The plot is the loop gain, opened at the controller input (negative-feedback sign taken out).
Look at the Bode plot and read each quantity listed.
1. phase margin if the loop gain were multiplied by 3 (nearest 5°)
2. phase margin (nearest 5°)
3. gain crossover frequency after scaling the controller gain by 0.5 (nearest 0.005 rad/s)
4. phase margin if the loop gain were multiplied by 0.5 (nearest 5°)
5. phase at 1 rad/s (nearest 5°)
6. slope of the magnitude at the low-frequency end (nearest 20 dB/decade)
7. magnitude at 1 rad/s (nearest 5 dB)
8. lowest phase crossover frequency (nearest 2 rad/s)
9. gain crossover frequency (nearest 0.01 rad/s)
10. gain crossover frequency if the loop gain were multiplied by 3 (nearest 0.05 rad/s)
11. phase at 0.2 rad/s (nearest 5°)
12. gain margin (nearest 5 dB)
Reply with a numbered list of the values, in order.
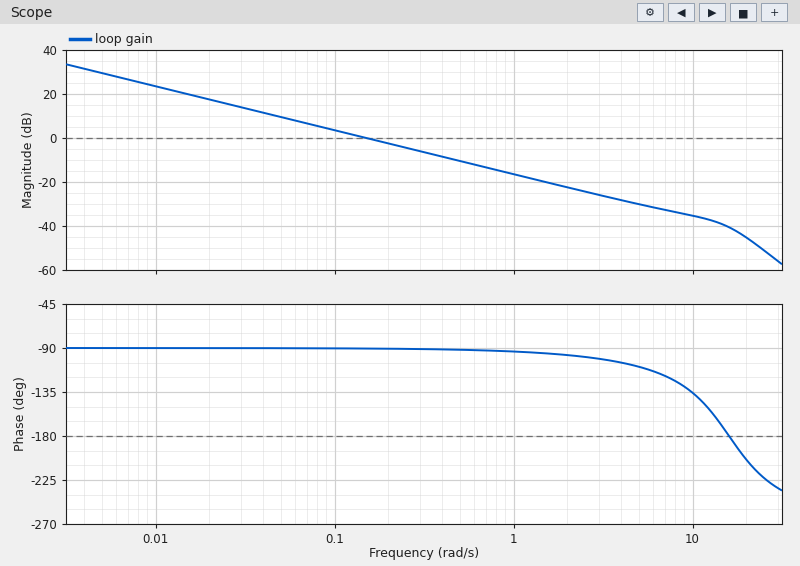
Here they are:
1. 90°
2. 90°
3. 0.075 rad/s
4. 90°
5. -95°
6. -20 dB/decade
7. -15 dB
8. 16 rad/s
9. 0.15 rad/s
10. 0.45 rad/s
11. -90°
12. 40 dB
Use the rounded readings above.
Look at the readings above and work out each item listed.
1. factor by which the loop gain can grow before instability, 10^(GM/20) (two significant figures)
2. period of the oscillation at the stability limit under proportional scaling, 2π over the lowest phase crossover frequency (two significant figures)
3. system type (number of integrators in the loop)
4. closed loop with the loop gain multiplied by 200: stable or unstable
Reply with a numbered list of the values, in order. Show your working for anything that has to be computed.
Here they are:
1. 10^(40 / 20) = 100
2. 2π / 16 = 0.39 s
3. 1
4. unstable
